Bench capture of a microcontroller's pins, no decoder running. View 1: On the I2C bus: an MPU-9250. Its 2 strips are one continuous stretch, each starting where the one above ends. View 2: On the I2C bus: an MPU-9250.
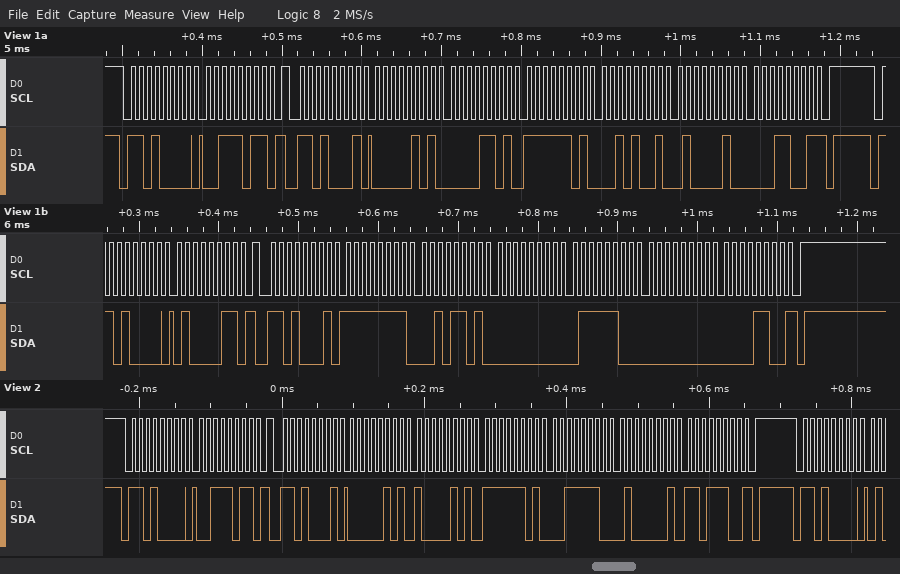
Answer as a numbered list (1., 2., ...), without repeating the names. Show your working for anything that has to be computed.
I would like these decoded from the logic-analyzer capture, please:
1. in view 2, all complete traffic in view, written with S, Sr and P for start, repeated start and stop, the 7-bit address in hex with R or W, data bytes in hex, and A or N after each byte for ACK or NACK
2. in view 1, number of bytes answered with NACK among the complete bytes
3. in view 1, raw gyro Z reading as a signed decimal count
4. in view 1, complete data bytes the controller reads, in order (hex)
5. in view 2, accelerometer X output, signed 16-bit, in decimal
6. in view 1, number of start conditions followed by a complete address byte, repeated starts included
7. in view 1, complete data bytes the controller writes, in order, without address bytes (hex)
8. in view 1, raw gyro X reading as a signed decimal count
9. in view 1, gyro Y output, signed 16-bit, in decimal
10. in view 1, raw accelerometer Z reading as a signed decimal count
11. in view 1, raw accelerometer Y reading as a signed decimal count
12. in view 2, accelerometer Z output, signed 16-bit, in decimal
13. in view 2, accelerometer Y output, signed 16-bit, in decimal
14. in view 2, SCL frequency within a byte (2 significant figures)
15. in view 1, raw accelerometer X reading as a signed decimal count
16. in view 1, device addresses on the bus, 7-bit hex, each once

1. S 68W A 3B A Sr 68R A 05 A 85 A FD A 3E A 41 A DC N P S 68W A
2. 2
3. 0x000C = 12
4. 05 0D FD 29 42 19 FF 2D 00 7C 00 0C
5. 0x0585 = 1413
6. 4
7. 3B 43
8. 0xFF2D = -211
9. 0x007C = 124
10. 0x4219 = 16921
11. 0xFD29 = -727
12. 0x41DC = 16860
13. 0xFD3E = -706
14. 100 kHz
15. 0x050D = 1293
16. 0x68
